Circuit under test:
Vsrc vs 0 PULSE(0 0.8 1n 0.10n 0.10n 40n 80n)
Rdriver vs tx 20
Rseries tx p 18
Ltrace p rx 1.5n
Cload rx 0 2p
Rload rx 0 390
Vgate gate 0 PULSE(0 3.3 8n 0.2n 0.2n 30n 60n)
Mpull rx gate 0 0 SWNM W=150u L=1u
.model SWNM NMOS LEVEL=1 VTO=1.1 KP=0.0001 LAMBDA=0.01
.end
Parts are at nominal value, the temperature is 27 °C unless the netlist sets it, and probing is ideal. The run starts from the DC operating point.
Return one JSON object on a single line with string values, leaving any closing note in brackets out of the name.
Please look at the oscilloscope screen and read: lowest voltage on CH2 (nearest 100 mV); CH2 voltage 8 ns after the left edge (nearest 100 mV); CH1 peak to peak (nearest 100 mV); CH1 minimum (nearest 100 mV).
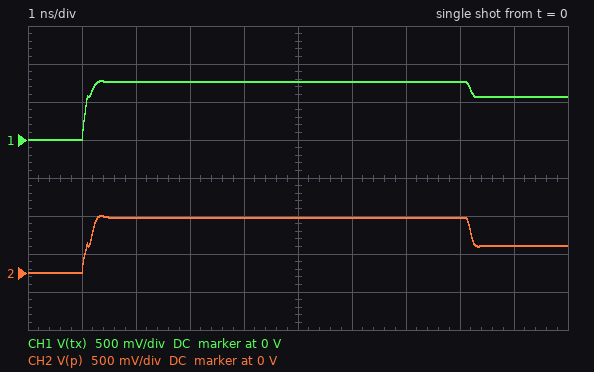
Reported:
{"lowest voltage on CH2": "0 V", "CH2 voltage 8 ns after the left edge": "700 mV", "CH1 peak to peak": "800 mV", "CH1 minimum": "0 V"}
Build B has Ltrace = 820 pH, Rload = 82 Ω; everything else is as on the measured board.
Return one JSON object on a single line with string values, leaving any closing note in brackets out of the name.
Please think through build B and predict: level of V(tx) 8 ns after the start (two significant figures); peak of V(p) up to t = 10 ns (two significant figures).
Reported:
{"level of V(tx) 8 ns after the start": "670 mV", "peak of V(p) up to t = 10 ns": "550 mV"}
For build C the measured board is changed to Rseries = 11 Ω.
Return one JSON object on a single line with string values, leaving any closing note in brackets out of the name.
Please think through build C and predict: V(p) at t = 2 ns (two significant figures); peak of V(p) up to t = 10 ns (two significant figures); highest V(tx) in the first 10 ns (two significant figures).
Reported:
{"V(p) at t = 2 ns": "740 mV", "peak of V(p) up to t = 10 ns": "780 mV", "highest V(tx) in the first 10 ns": "790 mV"}
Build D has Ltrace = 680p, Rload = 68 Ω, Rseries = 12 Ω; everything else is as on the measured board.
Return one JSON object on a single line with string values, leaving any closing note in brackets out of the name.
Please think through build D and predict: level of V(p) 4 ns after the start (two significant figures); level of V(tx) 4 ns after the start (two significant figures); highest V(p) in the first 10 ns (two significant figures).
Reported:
{"level of V(p) 4 ns after the start": "540 mV", "level of V(tx) 4 ns after the start": "640 mV", "highest V(p) in the first 10 ns": "550 mV"}
